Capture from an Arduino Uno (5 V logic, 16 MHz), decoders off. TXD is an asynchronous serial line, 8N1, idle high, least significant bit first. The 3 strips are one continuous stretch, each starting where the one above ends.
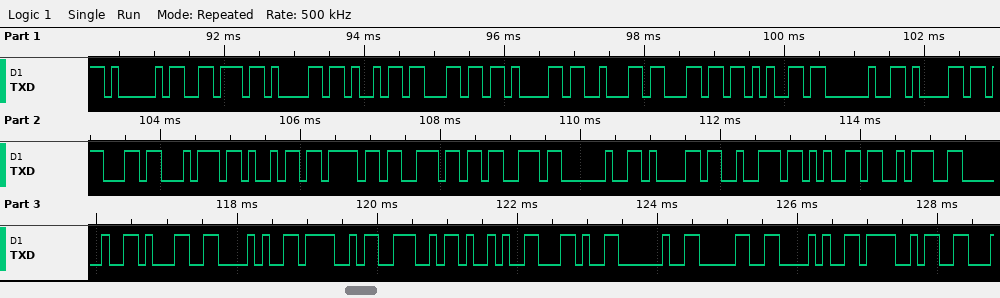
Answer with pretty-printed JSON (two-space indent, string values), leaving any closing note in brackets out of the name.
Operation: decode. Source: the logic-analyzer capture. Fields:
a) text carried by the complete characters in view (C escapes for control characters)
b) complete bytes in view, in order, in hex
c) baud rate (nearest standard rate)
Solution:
{
  "text carried by the complete characters in view": "\"Available actions are: 1(ON), 0(O\"",
  "complete bytes in view, in order, in hex": "41 76 61 69 6C 61 62 6C 65 20 61 63 74 69 6F 6E 73 20 61 72 65 3A 20 31 28 4F 4E 29 2C 20 30 28 4F",
  "baud rate": "9600 baud"
}
